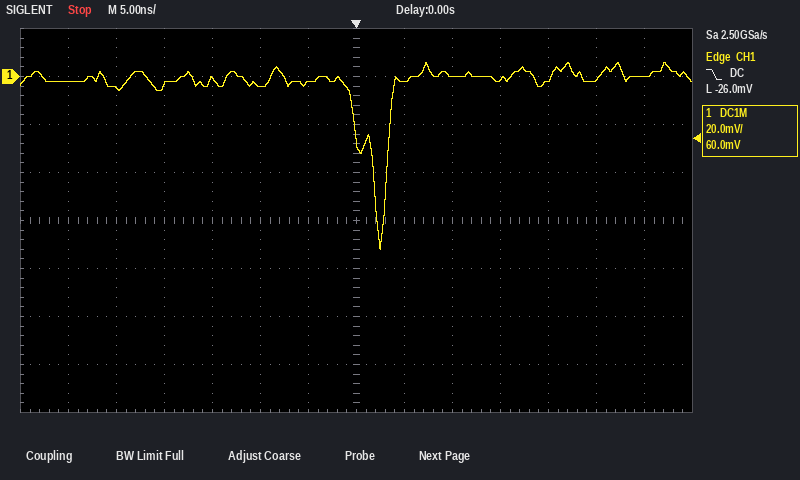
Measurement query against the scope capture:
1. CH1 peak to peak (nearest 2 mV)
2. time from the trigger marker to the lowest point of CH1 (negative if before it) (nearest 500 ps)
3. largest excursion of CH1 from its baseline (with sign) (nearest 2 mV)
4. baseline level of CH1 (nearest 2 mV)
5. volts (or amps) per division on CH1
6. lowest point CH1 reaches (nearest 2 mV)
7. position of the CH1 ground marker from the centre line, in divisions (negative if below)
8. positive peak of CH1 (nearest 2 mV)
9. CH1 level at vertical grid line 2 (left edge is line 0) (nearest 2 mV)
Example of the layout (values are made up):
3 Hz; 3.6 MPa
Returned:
78 mV; +2.5 ns; -72 mV; 0 mV; 20 mV; -72 mV; +3.0 div; 6 mV; -4 mV
